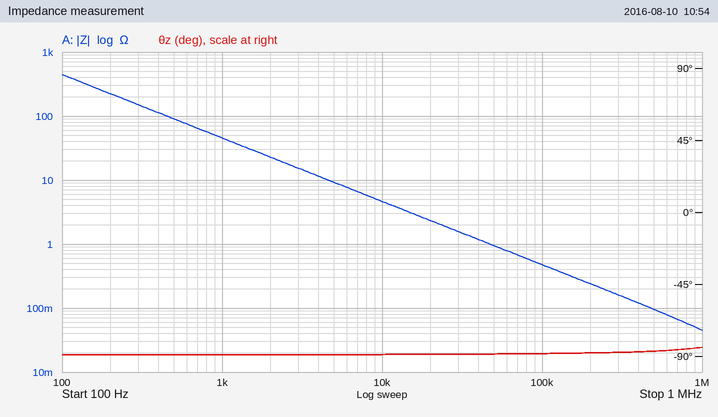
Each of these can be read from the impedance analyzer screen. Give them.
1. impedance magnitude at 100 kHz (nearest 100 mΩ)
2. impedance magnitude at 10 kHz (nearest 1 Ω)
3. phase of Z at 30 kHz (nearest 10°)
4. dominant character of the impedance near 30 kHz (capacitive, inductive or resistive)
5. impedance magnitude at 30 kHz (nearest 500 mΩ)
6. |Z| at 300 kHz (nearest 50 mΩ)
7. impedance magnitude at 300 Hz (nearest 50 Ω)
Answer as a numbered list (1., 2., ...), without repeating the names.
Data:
1. 500 mΩ
2. 5 Ω
3. -90°
4. capacitive
5. 1.5 Ω
6. 150 mΩ
7. 150 Ω
